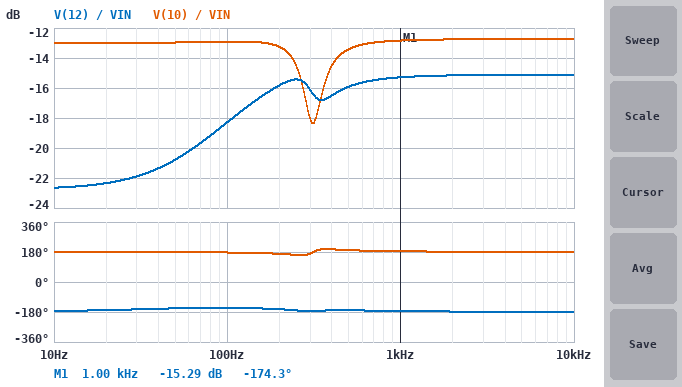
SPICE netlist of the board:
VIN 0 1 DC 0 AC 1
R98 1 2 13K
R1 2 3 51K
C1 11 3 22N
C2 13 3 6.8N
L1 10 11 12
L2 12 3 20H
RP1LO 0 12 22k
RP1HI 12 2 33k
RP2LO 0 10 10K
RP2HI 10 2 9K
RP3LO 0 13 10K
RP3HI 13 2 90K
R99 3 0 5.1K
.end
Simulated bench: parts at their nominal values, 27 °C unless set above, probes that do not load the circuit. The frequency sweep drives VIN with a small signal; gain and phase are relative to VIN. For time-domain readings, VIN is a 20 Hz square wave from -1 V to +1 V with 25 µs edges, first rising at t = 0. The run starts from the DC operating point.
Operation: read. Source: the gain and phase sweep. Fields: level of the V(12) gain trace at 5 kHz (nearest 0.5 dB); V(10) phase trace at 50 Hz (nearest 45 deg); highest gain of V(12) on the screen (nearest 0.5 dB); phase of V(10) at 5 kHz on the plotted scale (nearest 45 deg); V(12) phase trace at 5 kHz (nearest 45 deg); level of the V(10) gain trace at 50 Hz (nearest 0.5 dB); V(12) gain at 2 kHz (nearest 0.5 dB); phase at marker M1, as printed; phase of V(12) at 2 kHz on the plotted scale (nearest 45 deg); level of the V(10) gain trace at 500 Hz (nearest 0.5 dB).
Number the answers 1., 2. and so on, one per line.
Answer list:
1. -15.0 dB
2. 180 deg
3. -15.0 dB
4. 180 deg
5. -180 deg
6. -13.0 dB
7. -15.0 dB
8. -174.3 deg
9. -180 deg
10. -13.5 dB
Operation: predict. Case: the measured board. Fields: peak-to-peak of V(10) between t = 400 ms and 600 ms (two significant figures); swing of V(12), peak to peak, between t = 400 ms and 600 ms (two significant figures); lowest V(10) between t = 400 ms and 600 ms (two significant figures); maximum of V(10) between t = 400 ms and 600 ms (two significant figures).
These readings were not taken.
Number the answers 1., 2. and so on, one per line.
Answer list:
1. 530 mV
2. 550 mV
3. -260 mV
4. 260 mV
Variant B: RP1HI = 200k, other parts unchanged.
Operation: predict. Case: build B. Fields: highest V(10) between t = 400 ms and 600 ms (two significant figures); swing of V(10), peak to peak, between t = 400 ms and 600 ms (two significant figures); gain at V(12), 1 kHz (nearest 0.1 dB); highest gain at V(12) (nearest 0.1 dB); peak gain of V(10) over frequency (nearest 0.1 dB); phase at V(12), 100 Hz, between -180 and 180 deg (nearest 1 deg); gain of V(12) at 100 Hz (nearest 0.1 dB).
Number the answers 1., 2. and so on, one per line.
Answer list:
1. 290 mV
2. 580 mV
3. -26.9 dB
4. -22.1 dB
5. -12.0 dB
6. -170 deg
7. -25.7 dB
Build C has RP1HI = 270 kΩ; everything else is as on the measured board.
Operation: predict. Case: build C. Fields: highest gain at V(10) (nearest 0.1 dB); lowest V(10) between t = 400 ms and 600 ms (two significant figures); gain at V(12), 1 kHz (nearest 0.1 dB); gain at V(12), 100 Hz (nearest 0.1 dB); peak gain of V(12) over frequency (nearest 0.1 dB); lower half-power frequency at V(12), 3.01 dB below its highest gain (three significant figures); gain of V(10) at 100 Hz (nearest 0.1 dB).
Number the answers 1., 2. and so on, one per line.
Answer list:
1. -12.0 dB
2. -290 mV
3. -29.3 dB
4. -26.5 dB
5. -22.7 dB
6. 138 Hz
7. -12.1 dB
